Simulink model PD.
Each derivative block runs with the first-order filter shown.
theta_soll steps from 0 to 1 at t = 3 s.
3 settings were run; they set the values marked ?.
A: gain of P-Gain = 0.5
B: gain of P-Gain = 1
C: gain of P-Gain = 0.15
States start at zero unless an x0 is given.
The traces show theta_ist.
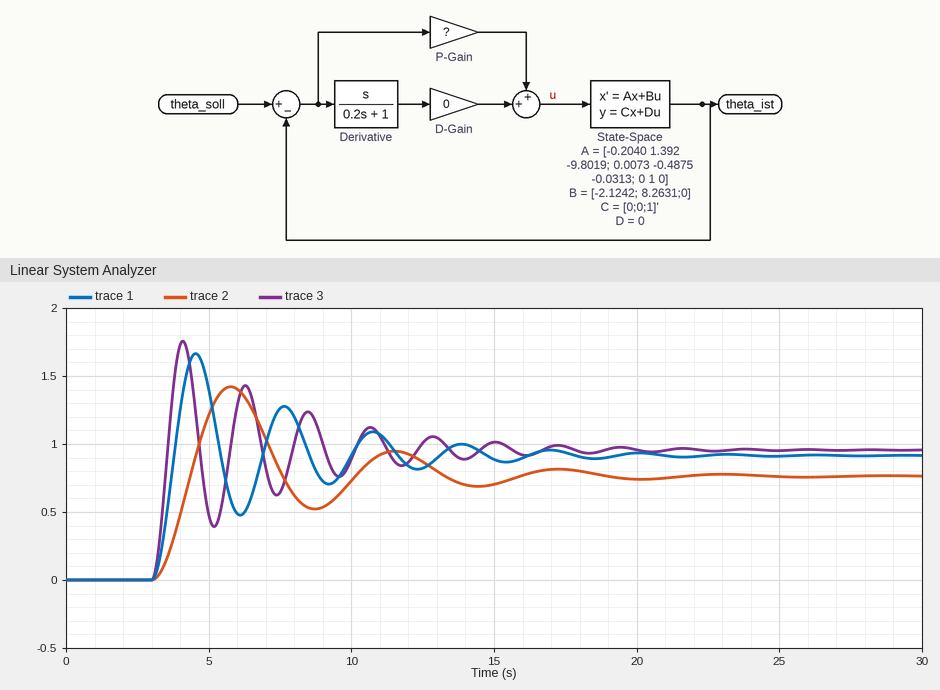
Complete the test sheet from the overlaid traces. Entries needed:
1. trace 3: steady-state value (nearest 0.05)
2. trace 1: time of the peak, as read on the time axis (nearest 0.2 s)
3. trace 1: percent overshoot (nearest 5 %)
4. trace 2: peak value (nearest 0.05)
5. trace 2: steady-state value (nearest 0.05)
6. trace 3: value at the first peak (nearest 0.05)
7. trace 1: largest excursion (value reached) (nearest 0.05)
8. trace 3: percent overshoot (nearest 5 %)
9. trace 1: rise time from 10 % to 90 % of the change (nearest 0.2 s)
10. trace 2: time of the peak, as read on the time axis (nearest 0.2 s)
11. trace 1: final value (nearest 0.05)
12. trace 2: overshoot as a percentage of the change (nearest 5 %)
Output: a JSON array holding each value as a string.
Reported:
["0.95", "4.6 s", "80 %", "1.40", "0.75", "1.75", "1.65", "85 %", "0.6 s", "5.8 s", "0.90", "85 %"]
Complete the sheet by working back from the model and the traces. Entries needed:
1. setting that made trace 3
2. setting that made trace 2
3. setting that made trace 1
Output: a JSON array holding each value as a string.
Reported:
["B", "C", "A"]
